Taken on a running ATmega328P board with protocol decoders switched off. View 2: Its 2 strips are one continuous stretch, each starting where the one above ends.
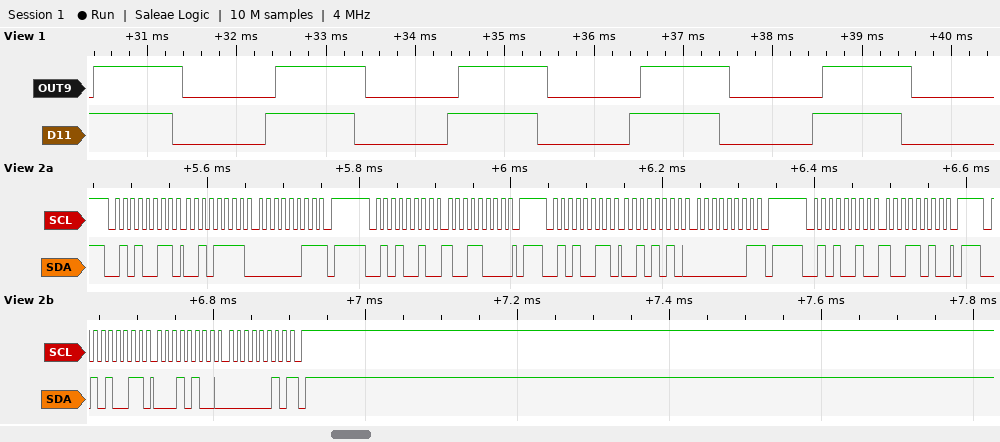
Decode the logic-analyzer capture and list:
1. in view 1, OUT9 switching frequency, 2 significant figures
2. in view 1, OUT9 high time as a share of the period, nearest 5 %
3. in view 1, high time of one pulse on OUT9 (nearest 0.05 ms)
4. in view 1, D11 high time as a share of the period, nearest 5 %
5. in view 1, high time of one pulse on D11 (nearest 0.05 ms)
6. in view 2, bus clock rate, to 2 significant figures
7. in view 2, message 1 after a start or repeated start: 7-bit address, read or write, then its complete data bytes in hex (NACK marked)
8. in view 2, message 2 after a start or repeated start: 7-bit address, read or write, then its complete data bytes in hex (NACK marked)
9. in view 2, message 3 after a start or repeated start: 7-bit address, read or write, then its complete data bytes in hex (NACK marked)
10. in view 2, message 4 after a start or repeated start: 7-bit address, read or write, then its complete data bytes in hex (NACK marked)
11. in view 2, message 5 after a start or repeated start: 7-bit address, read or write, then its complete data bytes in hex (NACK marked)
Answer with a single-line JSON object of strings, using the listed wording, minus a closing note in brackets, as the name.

{"in view 1, OUT9 switching frequency, 2 significant figures": "490 Hz", "in view 1, OUT9 high time as a share of the period, nearest 5 %": "50 %", "in view 1, high time of one pulse on OUT9": "1.00 ms", "in view 1, D11 high time as a share of the period, nearest 5 %": "50 %", "in view 1, high time of one pulse on D11": "1.00 ms", "in view 2, bus clock rate, to 2 significant figures": "100 kHz", "in view 2, message 1 after a start or repeated start: 7-bit address, read or write, then its complete data bytes in hex": "0x29 read: 2F 03 NACK", "in view 2, message 2 after a start or repeated start: 7-bit address, read or write, then its complete data bytes in hex": "0x29 write: 98", "in view 2, message 3 after a start or repeated start: 7-bit address, read or write, then its complete data bytes in hex": "0x29 read: 2A 01 NACK", "in view 2, message 4 after a start or repeated start: 7-bit address, read or write, then its complete data bytes in hex": "0x29 write: 9A", "in view 2, message 5 after a start or repeated start: 7-bit address, read or write, then its complete data bytes in hex": "0x29 read: 14 02 NACK"}
